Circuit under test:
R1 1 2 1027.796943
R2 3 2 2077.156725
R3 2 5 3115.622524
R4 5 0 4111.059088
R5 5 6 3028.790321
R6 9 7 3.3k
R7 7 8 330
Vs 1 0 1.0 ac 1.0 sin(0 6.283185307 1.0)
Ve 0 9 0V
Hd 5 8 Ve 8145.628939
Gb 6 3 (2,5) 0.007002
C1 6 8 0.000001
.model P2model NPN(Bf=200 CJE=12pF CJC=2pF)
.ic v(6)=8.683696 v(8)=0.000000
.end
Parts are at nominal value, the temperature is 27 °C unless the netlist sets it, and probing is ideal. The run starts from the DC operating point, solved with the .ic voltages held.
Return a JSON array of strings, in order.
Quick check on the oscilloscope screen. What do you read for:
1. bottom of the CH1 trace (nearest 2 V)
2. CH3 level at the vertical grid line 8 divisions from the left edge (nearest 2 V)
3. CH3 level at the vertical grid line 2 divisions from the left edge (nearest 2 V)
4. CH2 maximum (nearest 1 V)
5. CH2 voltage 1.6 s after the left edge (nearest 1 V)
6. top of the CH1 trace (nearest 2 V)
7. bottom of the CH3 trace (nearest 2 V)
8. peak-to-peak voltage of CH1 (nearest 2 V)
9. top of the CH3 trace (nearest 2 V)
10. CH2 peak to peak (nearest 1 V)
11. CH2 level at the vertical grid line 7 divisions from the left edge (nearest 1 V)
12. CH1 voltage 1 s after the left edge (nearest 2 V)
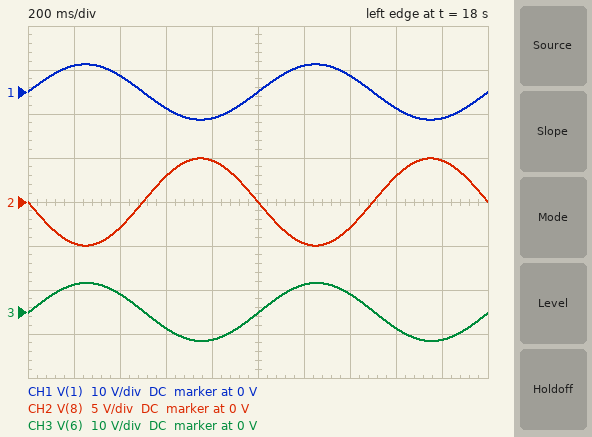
["-6 V", "-4 V", "4 V", "5 V", "3 V", "6 V", "-6 V", "12 V", "6 V", "10 V", "-3 V", "0 V"]
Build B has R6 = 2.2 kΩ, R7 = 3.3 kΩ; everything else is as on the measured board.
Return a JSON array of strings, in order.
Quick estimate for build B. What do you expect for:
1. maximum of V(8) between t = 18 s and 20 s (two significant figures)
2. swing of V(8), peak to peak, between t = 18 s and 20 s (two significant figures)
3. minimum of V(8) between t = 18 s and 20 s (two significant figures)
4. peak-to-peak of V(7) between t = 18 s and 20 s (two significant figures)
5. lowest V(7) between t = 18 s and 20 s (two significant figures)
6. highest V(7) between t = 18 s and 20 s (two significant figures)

["15 V", "30 V", "-15 V", "12 V", "-5.9 V", "5.9 V"]
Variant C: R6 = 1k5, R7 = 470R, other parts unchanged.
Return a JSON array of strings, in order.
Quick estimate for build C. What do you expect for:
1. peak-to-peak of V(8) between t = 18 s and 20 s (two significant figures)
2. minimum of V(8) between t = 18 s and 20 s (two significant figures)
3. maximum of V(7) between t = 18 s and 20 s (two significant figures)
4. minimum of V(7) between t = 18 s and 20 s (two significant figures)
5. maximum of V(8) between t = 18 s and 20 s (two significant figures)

["3.7 V", "-1.9 V", "1.4 V", "-1.4 V", "1.9 V"]
